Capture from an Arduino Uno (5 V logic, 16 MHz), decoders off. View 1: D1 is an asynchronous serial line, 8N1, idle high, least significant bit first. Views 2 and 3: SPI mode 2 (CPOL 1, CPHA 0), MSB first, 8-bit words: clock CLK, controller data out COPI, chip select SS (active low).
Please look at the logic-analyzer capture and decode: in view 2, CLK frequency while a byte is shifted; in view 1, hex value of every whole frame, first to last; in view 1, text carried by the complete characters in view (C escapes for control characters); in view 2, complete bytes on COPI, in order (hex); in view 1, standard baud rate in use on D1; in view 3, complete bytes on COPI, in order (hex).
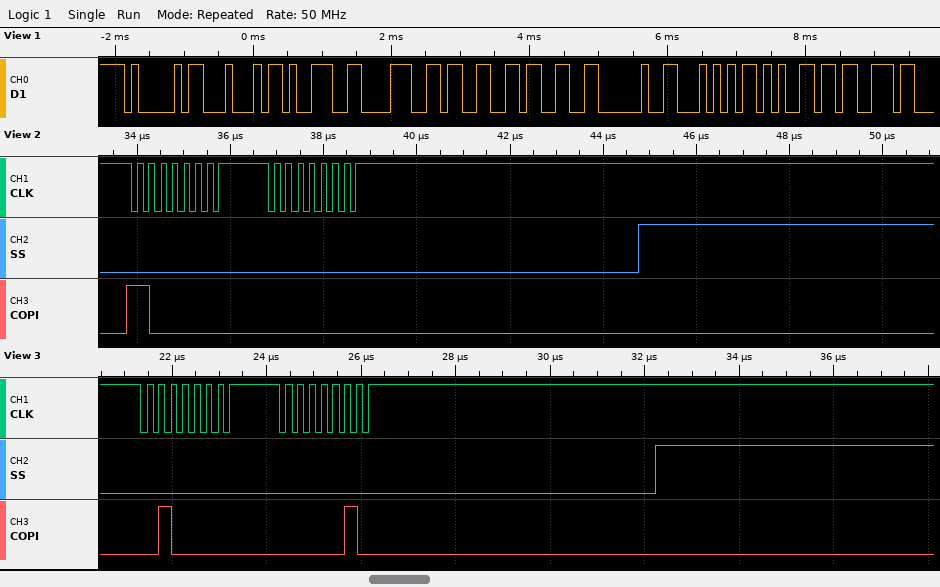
4 MHz
41 44 39 38 33 33 20 54 65 73
"AD9833 Tes"
C0 00
9600 baud
20 02
